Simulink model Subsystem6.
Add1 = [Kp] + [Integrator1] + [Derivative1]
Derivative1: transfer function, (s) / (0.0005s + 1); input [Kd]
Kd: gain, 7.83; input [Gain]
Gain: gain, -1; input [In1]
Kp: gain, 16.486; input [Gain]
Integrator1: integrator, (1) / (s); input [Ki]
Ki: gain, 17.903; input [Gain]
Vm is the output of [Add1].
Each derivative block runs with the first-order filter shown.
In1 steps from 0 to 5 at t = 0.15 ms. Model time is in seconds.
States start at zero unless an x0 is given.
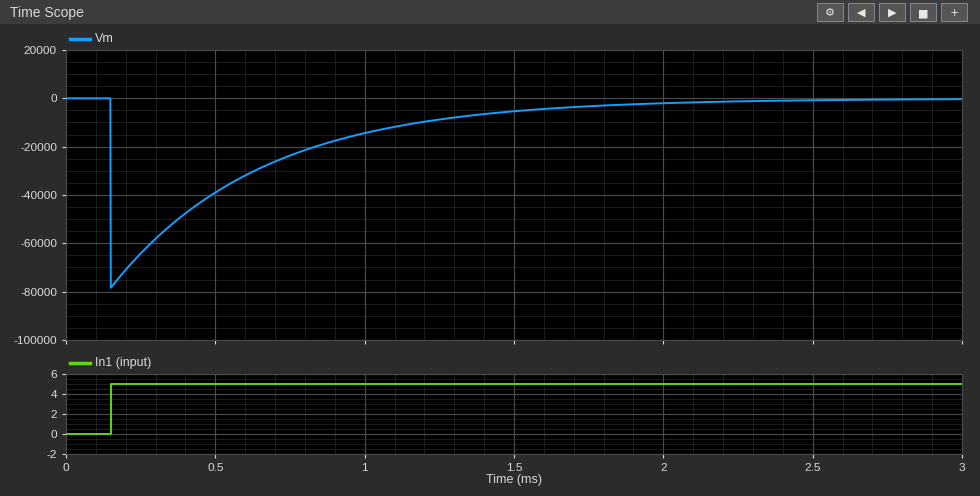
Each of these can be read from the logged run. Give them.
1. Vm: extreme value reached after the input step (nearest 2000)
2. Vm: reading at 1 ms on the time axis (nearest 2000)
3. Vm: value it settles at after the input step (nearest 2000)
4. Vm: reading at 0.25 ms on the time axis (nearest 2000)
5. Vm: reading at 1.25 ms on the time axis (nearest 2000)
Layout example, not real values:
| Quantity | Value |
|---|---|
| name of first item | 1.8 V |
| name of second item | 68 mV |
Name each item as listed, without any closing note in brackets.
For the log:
| Quantity | Value |
|---|---|
| Vm: extreme value reached after the input step | -78000 |
| Vm: reading at 1 ms on the time axis | -14000 |
| Vm: value it settles at after the input step | 0 |
| Vm: reading at 0.25 ms on the time axis | -64000 |
| Vm: reading at 1.25 ms on the time axis | -8000 |
